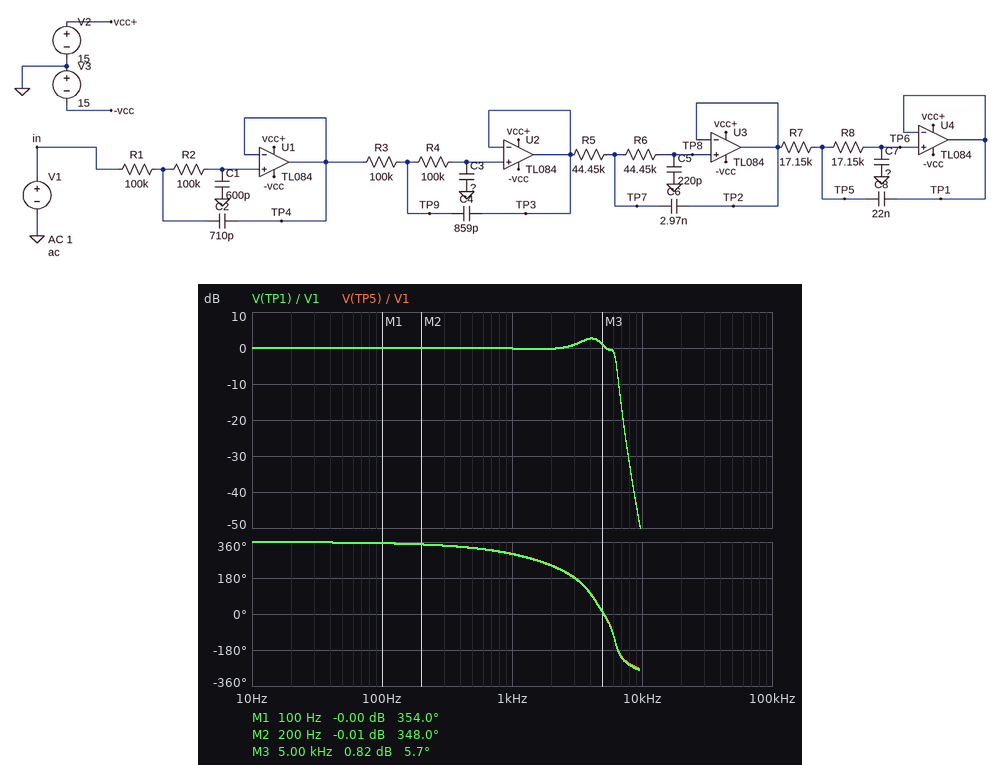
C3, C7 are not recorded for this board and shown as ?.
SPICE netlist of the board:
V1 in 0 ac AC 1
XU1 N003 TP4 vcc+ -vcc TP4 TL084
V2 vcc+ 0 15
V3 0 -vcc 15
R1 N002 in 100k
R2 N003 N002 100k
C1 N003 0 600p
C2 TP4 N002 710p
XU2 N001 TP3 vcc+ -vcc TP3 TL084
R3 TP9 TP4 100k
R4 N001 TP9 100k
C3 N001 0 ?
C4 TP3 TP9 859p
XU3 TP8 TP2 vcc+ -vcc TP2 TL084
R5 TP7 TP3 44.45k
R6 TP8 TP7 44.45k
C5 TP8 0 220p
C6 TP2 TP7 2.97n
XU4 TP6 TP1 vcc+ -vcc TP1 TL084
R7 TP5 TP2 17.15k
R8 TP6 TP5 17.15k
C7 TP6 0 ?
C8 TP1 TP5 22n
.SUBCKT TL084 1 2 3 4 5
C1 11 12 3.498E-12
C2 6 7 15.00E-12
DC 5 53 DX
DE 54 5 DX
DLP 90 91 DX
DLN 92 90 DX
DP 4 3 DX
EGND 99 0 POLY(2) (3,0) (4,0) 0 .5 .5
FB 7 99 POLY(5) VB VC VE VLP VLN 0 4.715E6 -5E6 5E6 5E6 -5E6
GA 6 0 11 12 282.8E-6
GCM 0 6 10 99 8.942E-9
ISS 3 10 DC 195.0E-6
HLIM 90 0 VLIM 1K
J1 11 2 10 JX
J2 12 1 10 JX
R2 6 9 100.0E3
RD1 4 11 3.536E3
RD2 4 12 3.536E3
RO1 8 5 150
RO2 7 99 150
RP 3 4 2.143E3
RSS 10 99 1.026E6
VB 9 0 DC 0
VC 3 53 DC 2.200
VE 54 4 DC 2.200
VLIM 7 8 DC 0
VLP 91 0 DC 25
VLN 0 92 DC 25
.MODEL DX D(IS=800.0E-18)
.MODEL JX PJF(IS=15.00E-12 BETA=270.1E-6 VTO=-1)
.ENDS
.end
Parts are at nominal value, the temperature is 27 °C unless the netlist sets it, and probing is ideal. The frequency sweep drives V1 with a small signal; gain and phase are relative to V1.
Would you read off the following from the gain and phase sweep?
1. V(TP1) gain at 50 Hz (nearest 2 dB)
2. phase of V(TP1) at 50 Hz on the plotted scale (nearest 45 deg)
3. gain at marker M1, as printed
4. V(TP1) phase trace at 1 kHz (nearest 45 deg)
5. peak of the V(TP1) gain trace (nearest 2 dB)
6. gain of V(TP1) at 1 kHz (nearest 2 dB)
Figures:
0 dB
360 deg
-0.00 dB
315 deg
2 dB
0 dB
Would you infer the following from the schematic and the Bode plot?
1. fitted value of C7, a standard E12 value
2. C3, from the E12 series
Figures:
100 pF
120 pF
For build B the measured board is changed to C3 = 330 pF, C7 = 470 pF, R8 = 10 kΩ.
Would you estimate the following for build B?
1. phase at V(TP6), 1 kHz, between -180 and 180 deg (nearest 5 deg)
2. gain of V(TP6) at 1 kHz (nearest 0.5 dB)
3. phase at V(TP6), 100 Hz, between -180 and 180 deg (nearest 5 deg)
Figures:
-80 deg
0 dB
-10 deg
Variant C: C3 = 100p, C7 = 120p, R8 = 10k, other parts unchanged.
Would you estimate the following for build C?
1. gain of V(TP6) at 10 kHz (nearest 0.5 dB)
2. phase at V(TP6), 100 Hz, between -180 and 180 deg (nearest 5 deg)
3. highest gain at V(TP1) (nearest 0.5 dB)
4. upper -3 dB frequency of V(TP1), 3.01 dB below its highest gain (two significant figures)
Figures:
-45.0 dB
-5 deg
1.0 dB
5.1 kHz
